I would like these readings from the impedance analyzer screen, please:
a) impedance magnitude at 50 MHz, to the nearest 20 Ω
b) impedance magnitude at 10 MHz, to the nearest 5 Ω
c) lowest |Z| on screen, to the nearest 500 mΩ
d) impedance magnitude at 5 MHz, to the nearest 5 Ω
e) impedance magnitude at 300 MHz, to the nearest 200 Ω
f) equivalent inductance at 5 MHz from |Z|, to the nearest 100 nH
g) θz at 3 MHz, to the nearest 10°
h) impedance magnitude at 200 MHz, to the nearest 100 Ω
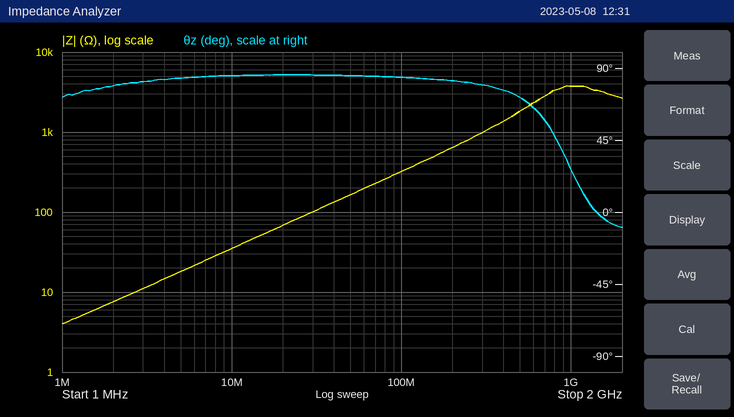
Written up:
160 Ω
35 Ω
4.0 Ω
20 Ω
1.0 kΩ
600 nH
80°
600 Ω
